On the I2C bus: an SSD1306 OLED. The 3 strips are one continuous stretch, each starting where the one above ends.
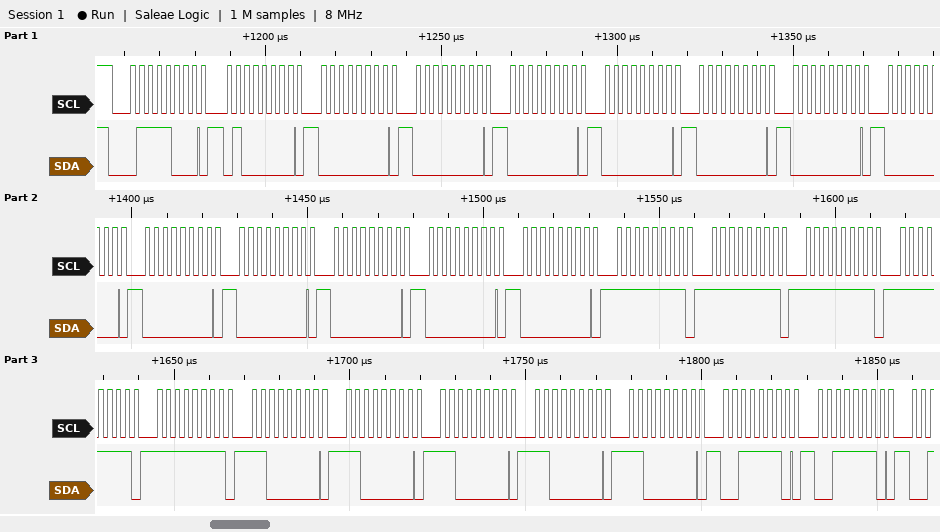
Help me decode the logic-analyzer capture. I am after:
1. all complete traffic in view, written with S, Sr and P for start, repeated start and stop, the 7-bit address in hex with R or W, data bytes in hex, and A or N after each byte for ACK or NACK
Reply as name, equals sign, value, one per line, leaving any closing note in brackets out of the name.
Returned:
all complete traffic in view, written with S, Sr and P for start, repeated start and stop, the 7-bit address in hex with R or W, data bytes in hex, and A or N after each byte for ACK or NACK = S 3CW A 40 A 00 A 00 A 00 A 00 A 00 A 00 A 00 A 00 A 00 A 00 A 00 A 00 A FF A FF A FF A FF A FF A C0 A C0 A C0 A C0 A C0 A 3E A 3E A
